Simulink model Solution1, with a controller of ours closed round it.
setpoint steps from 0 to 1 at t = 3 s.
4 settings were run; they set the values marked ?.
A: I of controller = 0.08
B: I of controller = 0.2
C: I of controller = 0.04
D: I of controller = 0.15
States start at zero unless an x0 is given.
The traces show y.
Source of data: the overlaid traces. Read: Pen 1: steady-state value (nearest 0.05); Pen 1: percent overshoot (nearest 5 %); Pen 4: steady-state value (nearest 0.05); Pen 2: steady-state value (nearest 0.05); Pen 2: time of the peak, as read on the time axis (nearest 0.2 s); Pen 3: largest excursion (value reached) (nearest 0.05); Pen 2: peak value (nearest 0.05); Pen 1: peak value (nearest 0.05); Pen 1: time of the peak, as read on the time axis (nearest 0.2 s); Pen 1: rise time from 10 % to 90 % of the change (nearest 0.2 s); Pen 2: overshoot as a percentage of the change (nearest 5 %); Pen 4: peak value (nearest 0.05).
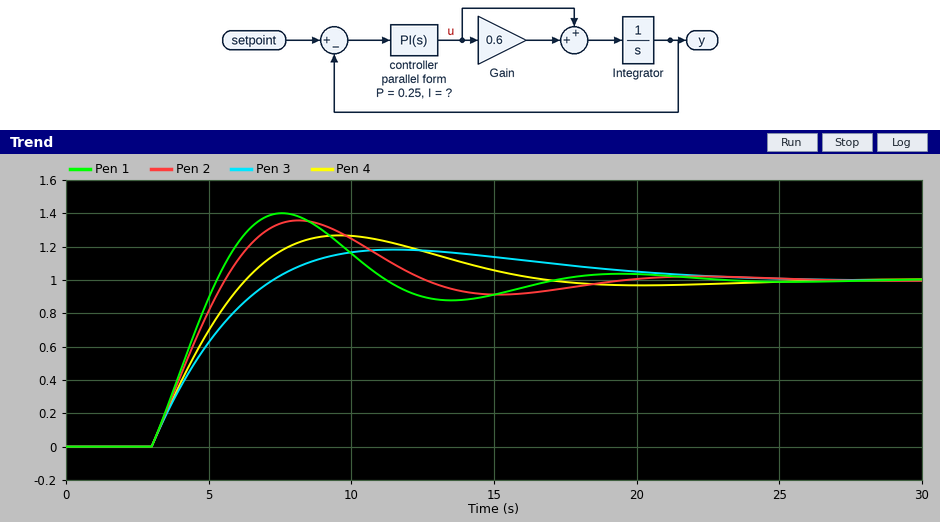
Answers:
1.00
40 %
1.00
1.00
8.2 s
1.20
1.35
1.40
7.6 s
1.8 s
35 %
1.25
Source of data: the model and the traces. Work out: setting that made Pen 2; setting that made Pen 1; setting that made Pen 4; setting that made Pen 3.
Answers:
D
B
A
C
